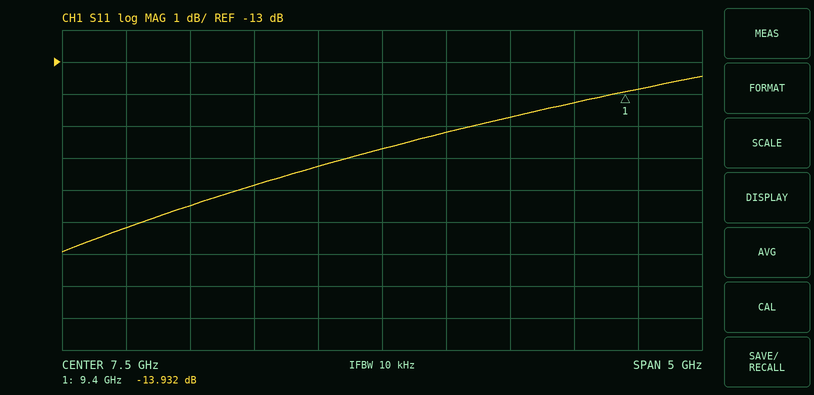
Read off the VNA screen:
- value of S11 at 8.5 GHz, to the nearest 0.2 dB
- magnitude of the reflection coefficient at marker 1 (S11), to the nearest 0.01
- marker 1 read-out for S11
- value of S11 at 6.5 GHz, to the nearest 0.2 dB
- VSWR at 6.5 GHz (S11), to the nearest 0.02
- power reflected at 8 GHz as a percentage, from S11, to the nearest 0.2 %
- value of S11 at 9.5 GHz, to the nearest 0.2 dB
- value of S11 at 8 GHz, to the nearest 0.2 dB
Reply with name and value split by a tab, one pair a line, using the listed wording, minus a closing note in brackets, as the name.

value of S11 at 8.5 GHz, to the nearest 0.2 dB	-14.8 dB
magnitude of the reflection coefficient at marker 1 (S11), to the nearest 0.01	0.20
marker 1 read-out for S11	-13.932 dB
value of S11 at 6.5 GHz, to the nearest 0.2 dB	-16.8 dB
VSWR at 6.5 GHz (S11), to the nearest 0.02	1.34
power reflected at 8 GHz as a percentage, from S11, to the nearest 0.2 %	3.0 %
value of S11 at 9.5 GHz, to the nearest 0.2 dB	-13.8 dB
value of S11 at 8 GHz, to the nearest 0.2 dB	-15.2 dB
